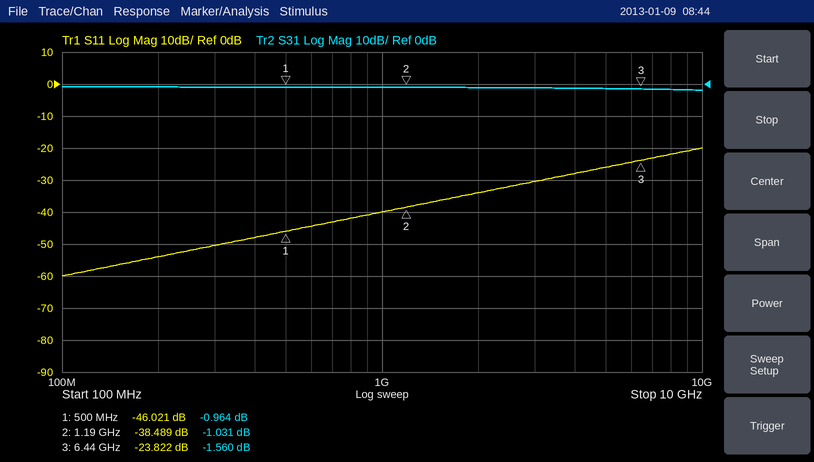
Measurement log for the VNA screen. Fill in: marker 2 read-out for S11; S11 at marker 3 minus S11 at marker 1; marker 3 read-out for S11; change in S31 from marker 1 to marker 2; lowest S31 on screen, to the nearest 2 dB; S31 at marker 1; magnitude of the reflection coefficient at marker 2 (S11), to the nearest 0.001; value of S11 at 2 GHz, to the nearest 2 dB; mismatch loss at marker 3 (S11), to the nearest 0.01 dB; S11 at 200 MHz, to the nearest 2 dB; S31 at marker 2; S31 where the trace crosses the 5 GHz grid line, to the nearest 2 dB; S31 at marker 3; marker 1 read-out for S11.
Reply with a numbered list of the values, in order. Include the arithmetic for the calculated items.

1. -38.489 dB
2. -23.822 − (-46.021) = 22.199 dB
3. -23.822 dB
4. -1.031 − (-0.964) = -0.067 dB
5. -2 dB
6. -0.964 dB
7. 10^(-38.489/20) ≈ 0.012
8. -34 dB
9. −10 log10(1 − 10^(-23.822/10)) ≈ 0.02 dB
10. -54 dB
11. -1.031 dB
12. -2 dB
13. -1.560 dB
14. -46.021 dB
